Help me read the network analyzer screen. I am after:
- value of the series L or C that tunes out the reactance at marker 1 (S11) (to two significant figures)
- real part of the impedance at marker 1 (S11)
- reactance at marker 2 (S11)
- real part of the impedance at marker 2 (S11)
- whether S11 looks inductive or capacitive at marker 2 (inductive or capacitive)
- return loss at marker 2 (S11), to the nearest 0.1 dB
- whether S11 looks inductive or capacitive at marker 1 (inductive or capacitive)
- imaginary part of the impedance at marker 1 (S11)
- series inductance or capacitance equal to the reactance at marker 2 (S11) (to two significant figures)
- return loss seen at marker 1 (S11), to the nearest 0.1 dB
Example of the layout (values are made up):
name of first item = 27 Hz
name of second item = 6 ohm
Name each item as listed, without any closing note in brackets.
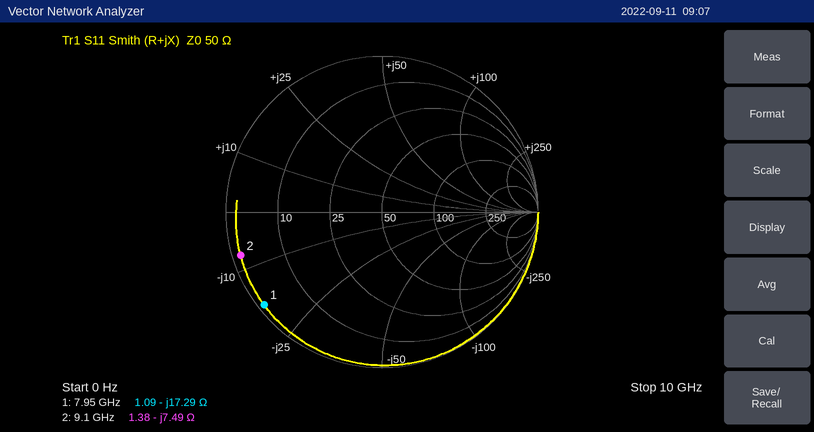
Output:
value of the series L or C that tunes out the reactance at marker 1 (S11) = 350 pH
real part of the impedance at marker 1 = 1.09 Ω
reactance at marker 2 = -7.49 Ω
real part of the impedance at marker 2 = 1.38 Ω
whether S11 looks inductive or capacitive at marker 2 = capacitive
return loss at marker 2 (S11), to the nearest 0.1 dB = 0.5 dB
whether S11 looks inductive or capacitive at marker 1 = capacitive
imaginary part of the impedance at marker 1 = -17.29 Ω
series inductance or capacitance equal to the reactance at marker 2 (S11) = 2.3 pF
return loss seen at marker 1 (S11), to the nearest 0.1 dB = 0.3 dB
